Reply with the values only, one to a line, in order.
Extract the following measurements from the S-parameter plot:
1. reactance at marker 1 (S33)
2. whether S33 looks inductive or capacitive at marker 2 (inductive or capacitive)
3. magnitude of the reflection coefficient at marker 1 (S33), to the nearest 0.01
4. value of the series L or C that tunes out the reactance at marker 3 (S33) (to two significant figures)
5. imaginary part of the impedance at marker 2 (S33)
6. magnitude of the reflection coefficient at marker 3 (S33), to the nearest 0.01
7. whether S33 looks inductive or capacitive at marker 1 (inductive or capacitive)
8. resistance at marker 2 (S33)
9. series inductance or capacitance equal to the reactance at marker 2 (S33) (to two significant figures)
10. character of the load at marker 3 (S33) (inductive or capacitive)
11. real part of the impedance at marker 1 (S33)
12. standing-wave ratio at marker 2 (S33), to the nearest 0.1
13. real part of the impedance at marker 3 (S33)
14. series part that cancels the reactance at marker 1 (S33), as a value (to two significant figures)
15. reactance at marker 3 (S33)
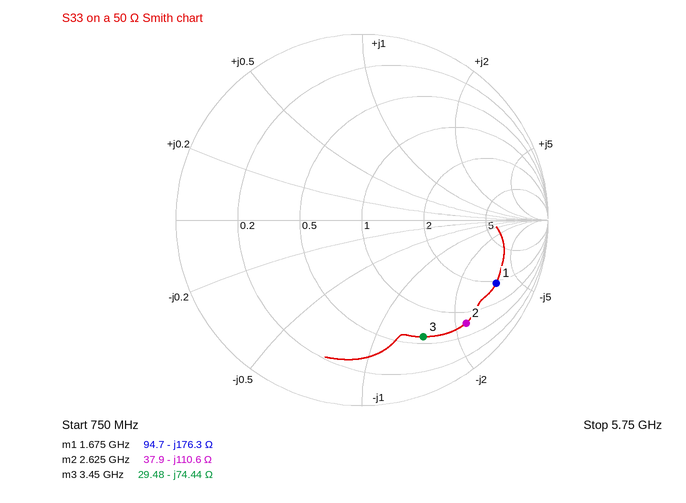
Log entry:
-176.3 Ω
capacitive
0.80
3.4 nH
-110.6 Ω
0.71
capacitive
37.9 Ω
550 fF
capacitive
94.7 Ω
8.4
29.48 Ω
17 nH
-74.44 Ω
